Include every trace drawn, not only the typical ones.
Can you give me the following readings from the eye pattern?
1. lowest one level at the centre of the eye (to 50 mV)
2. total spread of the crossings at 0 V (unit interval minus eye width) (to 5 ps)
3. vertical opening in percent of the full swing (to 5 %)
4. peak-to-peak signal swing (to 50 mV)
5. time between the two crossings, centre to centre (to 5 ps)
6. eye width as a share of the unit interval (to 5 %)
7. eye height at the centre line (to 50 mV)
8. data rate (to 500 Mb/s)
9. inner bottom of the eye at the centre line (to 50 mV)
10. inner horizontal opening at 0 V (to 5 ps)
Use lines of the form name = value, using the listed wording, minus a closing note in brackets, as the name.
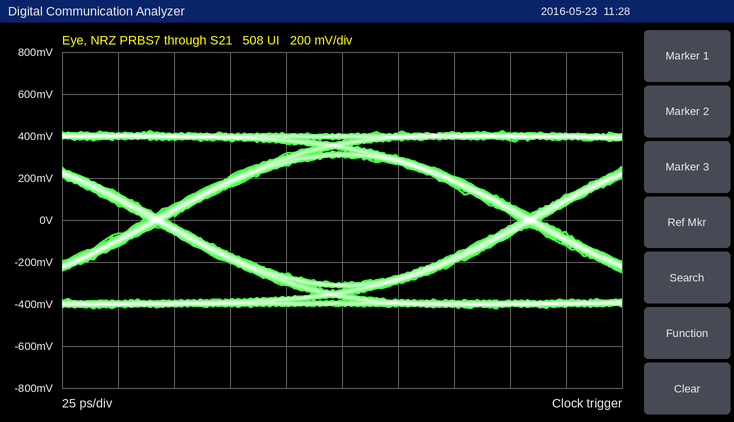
lowest one level at the centre of the eye = 300 mV
total spread of the crossings at 0 V (unit interval minus eye width) = 10 ps
vertical opening in percent of the full swing = 70 %
peak-to-peak signal swing = 850 mV
time between the two crossings, centre to centre = 165 ps
eye width as a share of the unit interval = 95 %
eye height at the centre line = 600 mV
data rate = 6.0 Gb/s
inner bottom of the eye at the centre line = -300 mV
inner horizontal opening at 0 V = 155 ps
